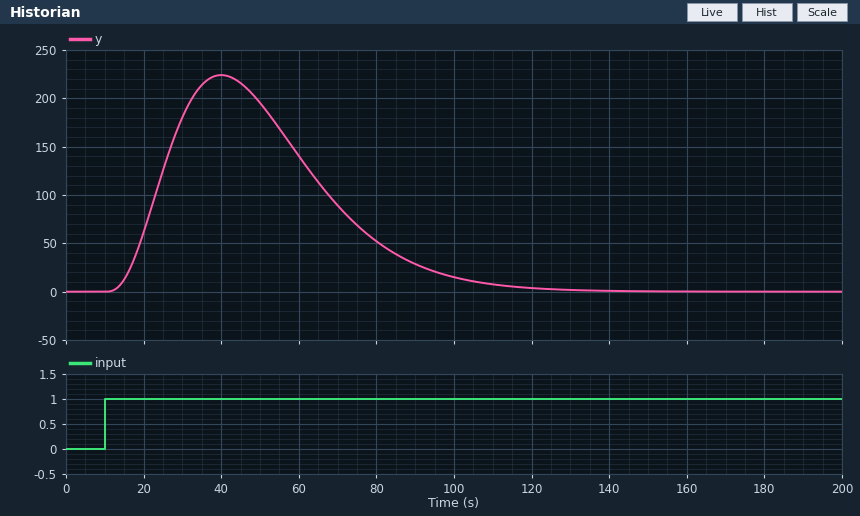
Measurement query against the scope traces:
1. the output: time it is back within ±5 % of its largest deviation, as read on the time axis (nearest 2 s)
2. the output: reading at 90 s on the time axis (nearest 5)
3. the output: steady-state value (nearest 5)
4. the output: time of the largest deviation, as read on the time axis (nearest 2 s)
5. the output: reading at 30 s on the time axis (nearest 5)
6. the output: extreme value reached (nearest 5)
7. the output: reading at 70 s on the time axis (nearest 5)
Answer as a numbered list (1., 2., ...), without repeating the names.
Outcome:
1. 104 s
2. 30
3. 0
4. 40 s
5. 180
6. 225
7. 90
